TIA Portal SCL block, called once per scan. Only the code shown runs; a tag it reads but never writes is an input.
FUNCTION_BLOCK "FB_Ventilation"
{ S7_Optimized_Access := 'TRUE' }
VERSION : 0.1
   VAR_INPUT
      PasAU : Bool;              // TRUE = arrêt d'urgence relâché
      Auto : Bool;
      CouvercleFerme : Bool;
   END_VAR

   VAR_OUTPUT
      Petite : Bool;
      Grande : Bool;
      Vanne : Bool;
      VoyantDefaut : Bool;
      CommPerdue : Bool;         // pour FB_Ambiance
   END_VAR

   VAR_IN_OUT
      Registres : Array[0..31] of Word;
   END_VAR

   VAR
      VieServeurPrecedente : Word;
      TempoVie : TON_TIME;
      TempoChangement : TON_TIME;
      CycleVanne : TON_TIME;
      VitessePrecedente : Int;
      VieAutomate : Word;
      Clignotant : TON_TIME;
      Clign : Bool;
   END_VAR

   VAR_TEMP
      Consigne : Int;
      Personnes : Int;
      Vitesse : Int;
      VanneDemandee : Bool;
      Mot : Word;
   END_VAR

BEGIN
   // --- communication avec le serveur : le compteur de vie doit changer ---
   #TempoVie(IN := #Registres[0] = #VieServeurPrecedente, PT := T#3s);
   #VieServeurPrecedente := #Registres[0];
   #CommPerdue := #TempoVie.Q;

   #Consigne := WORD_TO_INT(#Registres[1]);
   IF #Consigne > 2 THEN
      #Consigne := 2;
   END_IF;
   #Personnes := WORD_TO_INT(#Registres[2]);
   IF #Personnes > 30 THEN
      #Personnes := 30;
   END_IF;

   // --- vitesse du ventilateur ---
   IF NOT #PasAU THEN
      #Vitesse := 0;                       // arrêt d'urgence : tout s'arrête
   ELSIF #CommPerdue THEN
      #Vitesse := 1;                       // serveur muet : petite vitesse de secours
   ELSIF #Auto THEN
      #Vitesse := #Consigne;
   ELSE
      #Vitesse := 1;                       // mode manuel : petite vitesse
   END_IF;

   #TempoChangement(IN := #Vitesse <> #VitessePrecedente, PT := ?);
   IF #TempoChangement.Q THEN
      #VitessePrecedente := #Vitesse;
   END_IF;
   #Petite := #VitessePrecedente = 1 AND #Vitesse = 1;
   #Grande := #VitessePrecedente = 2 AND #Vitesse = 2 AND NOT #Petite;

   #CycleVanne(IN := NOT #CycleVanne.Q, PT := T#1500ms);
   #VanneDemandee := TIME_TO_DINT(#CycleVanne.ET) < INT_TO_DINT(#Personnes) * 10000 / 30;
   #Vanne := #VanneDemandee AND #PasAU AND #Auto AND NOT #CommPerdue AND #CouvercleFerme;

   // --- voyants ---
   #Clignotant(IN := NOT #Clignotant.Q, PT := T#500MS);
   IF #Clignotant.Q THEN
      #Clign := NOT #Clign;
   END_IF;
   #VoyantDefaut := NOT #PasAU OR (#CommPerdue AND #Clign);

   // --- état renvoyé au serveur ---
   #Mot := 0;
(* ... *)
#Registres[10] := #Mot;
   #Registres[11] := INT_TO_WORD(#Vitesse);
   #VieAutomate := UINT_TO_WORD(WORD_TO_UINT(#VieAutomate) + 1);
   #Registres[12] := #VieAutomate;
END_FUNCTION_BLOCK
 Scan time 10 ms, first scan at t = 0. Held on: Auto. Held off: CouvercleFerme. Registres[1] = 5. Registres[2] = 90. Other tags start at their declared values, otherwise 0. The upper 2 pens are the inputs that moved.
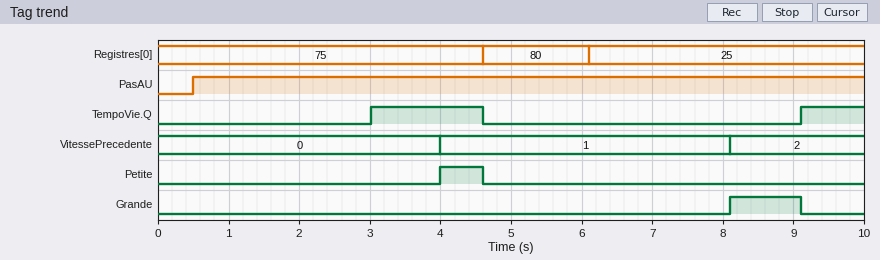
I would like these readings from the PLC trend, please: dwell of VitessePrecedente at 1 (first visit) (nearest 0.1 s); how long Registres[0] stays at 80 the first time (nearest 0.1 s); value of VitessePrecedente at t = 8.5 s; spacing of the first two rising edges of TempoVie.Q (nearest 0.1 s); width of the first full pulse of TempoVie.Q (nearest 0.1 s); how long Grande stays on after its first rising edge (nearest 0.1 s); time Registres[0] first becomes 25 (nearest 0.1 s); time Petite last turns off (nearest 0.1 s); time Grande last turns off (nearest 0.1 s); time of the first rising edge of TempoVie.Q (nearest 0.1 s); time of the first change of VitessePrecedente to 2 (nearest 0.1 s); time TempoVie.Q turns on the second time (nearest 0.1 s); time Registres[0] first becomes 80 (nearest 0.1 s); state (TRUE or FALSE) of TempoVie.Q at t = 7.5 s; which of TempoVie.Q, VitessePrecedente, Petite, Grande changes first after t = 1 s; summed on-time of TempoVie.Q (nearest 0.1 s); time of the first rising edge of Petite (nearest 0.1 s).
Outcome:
4.1 s
1.5 s
2
6.1 s
1.6 s
1.0 s
6.1 s
4.6 s
9.1 s
3.0 s
8.1 s
9.1 s
4.6 s
FALSE
TempoVie.Q
2.5 s
4.0 s
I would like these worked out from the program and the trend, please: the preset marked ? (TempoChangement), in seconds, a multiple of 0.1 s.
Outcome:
3.5 s
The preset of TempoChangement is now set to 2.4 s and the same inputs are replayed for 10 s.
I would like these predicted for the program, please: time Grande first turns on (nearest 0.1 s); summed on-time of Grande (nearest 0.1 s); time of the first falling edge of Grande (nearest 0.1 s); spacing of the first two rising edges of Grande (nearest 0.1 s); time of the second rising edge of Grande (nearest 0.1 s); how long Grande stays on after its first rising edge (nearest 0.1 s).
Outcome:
2.9 s
4.6 s
3.0 s
1.7 s
4.6 s
0.1 s
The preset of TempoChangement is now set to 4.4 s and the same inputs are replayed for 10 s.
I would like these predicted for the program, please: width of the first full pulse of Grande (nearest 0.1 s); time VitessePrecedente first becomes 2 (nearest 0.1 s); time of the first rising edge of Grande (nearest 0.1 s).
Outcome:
4.2 s
4.9 s
4.9 s
